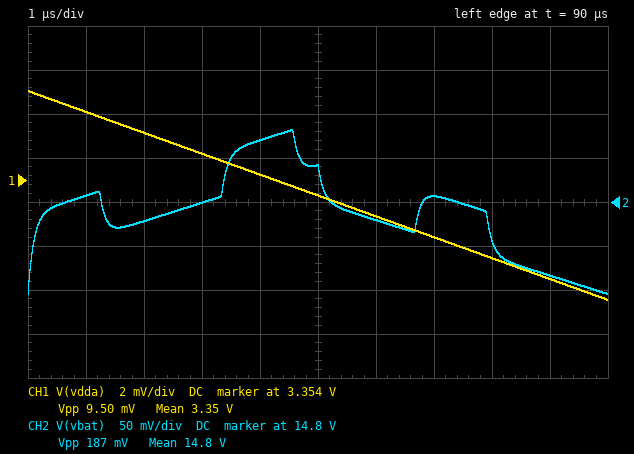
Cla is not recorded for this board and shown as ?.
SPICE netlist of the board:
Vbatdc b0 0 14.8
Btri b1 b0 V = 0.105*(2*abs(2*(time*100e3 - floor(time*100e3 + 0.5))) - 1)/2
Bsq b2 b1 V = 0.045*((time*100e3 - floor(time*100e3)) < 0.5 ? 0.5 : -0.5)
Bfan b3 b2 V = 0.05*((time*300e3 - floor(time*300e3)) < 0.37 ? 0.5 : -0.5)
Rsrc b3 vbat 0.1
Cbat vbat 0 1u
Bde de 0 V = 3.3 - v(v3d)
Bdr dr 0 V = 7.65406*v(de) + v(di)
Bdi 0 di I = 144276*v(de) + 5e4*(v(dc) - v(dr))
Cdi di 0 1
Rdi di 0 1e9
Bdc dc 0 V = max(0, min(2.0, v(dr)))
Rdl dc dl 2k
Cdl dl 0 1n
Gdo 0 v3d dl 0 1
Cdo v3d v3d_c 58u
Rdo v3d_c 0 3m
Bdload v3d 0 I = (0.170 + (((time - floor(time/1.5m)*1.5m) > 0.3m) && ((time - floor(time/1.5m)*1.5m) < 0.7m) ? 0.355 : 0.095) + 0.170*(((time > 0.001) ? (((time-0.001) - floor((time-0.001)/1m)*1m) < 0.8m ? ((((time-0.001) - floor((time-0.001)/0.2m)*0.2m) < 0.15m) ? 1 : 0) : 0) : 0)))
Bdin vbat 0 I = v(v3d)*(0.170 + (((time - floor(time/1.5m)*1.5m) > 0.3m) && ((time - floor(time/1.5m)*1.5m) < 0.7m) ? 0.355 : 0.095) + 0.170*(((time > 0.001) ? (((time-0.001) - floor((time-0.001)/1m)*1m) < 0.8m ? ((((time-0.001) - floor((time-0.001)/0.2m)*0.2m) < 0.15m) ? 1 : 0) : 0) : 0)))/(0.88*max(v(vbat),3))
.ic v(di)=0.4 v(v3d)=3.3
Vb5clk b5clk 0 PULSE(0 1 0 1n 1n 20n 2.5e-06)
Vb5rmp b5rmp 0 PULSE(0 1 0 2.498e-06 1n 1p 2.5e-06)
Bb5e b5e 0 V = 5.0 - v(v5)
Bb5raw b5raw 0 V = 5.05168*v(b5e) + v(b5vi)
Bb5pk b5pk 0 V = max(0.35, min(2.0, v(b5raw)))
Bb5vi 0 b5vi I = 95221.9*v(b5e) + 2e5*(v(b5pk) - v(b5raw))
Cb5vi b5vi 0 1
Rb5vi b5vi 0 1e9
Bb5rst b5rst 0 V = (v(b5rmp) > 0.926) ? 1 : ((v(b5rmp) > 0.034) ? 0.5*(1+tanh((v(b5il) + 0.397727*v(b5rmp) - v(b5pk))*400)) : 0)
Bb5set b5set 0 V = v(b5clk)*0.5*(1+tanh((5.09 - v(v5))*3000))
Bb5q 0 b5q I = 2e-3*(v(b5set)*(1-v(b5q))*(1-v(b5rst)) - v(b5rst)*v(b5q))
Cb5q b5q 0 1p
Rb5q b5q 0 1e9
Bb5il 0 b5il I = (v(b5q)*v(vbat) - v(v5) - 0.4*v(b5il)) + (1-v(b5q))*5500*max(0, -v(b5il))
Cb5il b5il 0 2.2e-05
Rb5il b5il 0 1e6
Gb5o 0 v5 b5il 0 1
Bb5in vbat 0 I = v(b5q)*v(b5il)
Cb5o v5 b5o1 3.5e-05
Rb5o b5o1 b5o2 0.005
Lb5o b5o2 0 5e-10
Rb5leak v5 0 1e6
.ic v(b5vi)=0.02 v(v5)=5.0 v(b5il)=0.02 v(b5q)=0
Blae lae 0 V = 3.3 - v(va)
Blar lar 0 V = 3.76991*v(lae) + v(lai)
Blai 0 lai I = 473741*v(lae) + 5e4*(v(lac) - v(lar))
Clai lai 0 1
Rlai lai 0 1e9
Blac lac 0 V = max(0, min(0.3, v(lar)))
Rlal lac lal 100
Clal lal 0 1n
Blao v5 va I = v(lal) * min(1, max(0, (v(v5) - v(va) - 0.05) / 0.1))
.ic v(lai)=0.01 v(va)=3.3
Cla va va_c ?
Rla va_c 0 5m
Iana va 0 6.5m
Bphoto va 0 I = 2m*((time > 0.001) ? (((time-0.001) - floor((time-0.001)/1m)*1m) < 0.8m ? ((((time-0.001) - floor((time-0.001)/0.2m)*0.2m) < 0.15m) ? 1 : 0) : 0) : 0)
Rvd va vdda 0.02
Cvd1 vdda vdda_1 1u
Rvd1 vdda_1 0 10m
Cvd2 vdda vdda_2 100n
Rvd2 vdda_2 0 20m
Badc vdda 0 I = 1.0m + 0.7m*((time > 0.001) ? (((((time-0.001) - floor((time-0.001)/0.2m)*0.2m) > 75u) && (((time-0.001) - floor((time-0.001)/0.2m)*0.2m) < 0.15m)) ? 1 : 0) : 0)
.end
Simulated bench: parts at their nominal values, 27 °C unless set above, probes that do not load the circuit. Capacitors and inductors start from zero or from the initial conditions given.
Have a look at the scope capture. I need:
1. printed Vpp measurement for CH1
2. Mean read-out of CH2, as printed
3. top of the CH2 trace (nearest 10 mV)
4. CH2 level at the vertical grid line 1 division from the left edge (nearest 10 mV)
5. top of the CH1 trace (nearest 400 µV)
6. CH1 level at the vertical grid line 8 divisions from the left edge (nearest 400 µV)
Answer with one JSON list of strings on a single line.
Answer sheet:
["9.50 mV", "14.8 V", "14.88 V", "14.81 V", "3.3580 V", "3.3504 V"]
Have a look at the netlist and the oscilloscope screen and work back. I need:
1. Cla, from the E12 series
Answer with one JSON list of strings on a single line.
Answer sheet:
["6.8 µF"]
